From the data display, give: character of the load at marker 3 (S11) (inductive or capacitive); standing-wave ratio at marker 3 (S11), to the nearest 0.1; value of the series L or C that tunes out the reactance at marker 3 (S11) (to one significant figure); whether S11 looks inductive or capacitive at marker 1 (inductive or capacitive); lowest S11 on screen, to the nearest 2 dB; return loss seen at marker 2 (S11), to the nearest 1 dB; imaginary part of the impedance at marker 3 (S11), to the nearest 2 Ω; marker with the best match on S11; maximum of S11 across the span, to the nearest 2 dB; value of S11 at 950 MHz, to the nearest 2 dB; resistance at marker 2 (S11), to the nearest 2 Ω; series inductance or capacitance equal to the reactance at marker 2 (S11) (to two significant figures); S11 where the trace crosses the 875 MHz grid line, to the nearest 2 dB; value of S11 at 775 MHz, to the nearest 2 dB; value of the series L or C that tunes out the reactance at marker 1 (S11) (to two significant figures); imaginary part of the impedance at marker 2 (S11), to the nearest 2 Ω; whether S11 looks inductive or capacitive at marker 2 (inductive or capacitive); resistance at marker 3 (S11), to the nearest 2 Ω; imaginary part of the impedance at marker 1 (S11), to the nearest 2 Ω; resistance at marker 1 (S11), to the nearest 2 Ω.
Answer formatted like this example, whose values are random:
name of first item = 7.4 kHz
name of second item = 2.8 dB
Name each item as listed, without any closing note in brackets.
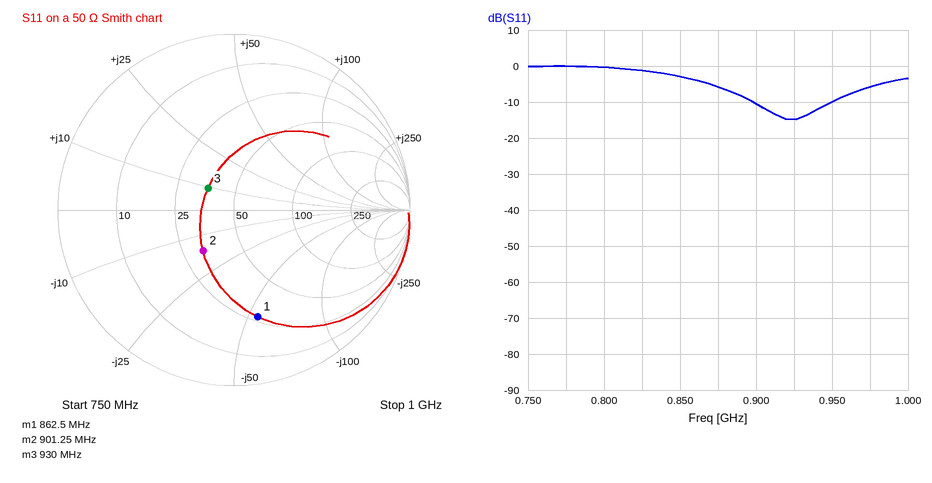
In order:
character of the load at marker 3 (S11) = inductive
standing-wave ratio at marker 3 (S11), to the nearest 0.1 = 1.5
value of the series L or C that tunes out the reactance at marker 3 (S11) = 20 pF
whether S11 looks inductive or capacitive at marker 1 = capacitive
lowest S11 on screen, to the nearest 2 dB = -14 dB
return loss seen at marker 2 (S11), to the nearest 1 dB = 11 dB
imaginary part of the impedance at marker 3 (S11), to the nearest 2 Ω = +10 Ω
marker with the best match on S11 = marker 3
maximum of S11 across the span, to the nearest 2 dB = 0 dB
value of S11 at 950 MHz, to the nearest 2 dB = -10 dB
resistance at marker 2 (S11), to the nearest 2 Ω = 32 Ω
series inductance or capacitance equal to the reactance at marker 2 (S11) = 11 pF
S11 where the trace crosses the 875 MHz grid line, to the nearest 2 dB = -6 dB
value of S11 at 775 MHz, to the nearest 2 dB = 0 dB
value of the series L or C that tunes out the reactance at marker 1 (S11) = 10 nH
imaginary part of the impedance at marker 2 (S11), to the nearest 2 Ω = -16 Ω
whether S11 looks inductive or capacitive at marker 2 = capacitive
resistance at marker 3 (S11), to the nearest 2 Ω = 36 Ω
imaginary part of the impedance at marker 1 (S11), to the nearest 2 Ω = -54 Ω
resistance at marker 1 (S11), to the nearest 2 Ω = 28 Ω
